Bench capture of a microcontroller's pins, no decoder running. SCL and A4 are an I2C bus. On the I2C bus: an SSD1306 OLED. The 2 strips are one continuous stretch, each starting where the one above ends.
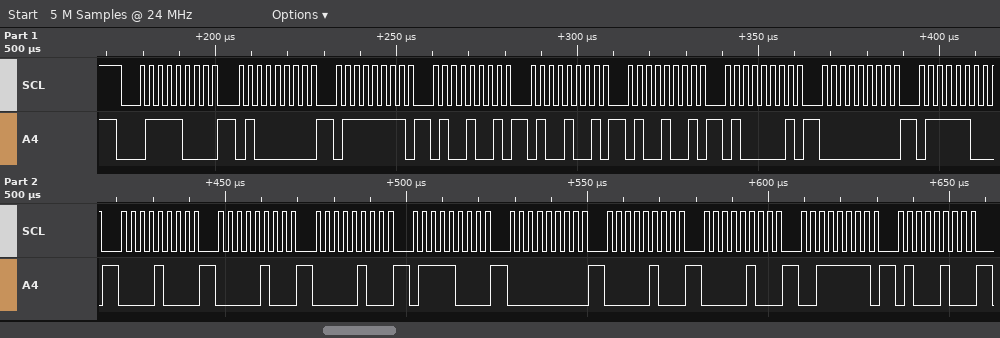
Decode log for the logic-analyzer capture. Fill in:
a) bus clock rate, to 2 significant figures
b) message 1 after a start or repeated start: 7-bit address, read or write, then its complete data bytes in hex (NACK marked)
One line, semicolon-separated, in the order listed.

400 kHz; 0x3C write: 40 7F 49 49 49 41 00 7C 08 04 04 78 00 04 04 3F 44
